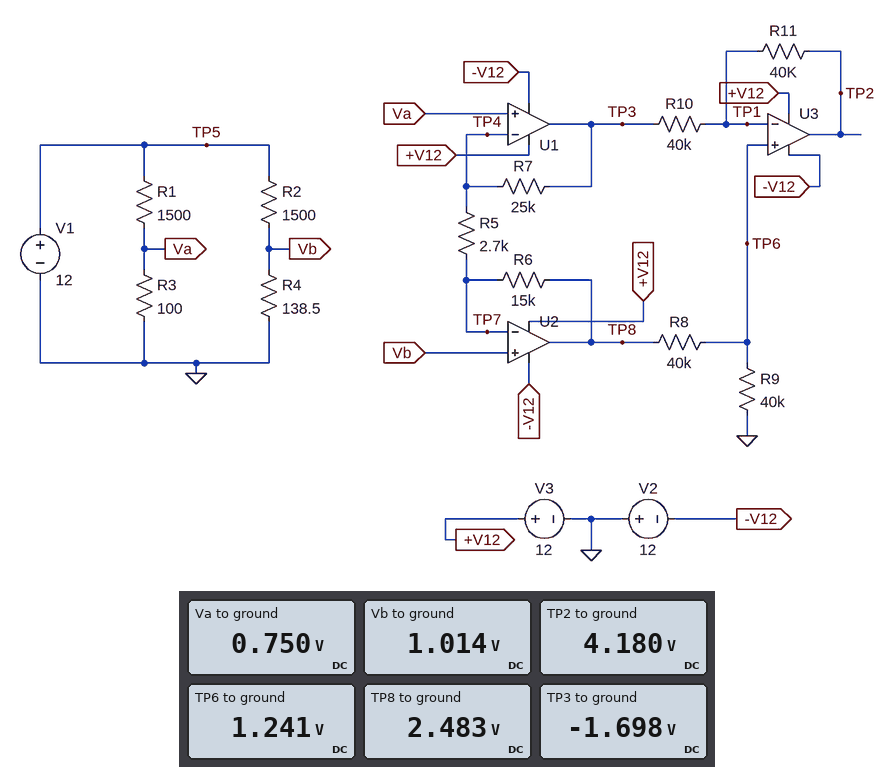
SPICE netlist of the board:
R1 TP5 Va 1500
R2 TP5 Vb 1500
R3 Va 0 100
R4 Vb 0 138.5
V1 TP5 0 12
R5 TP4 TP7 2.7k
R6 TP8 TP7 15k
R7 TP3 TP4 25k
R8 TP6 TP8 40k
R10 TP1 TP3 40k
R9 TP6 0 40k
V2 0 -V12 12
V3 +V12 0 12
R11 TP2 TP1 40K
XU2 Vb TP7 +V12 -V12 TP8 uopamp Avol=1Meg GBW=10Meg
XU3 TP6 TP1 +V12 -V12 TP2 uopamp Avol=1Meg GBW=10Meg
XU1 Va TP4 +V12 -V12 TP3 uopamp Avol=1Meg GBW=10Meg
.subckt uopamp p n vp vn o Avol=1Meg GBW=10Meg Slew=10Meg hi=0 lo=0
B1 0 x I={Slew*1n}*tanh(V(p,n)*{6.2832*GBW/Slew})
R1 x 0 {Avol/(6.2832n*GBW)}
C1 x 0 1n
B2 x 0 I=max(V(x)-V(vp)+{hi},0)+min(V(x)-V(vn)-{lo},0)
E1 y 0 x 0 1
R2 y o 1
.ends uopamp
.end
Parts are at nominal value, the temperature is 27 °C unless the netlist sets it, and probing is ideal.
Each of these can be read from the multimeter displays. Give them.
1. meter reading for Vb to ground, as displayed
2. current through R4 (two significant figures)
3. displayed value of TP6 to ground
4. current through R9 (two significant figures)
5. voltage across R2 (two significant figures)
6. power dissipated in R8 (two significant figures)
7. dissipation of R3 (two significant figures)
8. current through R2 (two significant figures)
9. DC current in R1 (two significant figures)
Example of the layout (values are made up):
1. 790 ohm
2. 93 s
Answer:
1. 1.014 V
2. 7.3 mA
3. 1.241 V
4. 31 µA
5. 11 V
6. 39 µW
7. 5.6 mW
8. 7.3 mA
9. 7.5 mA
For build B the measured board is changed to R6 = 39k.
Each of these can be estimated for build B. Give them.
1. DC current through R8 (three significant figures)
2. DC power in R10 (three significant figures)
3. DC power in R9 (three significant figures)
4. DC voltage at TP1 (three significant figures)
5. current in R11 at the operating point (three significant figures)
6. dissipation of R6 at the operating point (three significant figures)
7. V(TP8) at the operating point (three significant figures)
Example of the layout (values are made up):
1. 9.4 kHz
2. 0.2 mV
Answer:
1. 60.4 µA
2. 423 µW
3. 146 µW
4. 2.42 V
5. 103 µA
6. 374 µW
7. 4.83 V
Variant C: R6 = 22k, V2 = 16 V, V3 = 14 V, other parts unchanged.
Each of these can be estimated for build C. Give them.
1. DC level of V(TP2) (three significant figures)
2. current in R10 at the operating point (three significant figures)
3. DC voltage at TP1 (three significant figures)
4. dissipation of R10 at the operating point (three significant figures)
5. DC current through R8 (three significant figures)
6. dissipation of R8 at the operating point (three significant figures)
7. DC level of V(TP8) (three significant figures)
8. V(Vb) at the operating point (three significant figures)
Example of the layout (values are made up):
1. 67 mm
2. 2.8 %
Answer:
1. 4.87 V
2. 82.0 µA
3. 1.58 V
4. 269 µW
5. 39.6 µA
6. 62.7 µW
7. 3.17 V
8. 1.01 V
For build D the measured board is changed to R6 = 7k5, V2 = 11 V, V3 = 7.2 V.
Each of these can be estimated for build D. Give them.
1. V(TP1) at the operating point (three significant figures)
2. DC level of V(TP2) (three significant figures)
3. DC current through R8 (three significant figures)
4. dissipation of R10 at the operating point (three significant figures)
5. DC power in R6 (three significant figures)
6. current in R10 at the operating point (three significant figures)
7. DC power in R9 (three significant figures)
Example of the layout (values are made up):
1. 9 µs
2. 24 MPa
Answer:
1. 874 mV
2. 3.45 V
3. 21.9 µA
4. 165 µW
5. 71.9 µW
6. 64.3 µA
7. 19.1 µW
